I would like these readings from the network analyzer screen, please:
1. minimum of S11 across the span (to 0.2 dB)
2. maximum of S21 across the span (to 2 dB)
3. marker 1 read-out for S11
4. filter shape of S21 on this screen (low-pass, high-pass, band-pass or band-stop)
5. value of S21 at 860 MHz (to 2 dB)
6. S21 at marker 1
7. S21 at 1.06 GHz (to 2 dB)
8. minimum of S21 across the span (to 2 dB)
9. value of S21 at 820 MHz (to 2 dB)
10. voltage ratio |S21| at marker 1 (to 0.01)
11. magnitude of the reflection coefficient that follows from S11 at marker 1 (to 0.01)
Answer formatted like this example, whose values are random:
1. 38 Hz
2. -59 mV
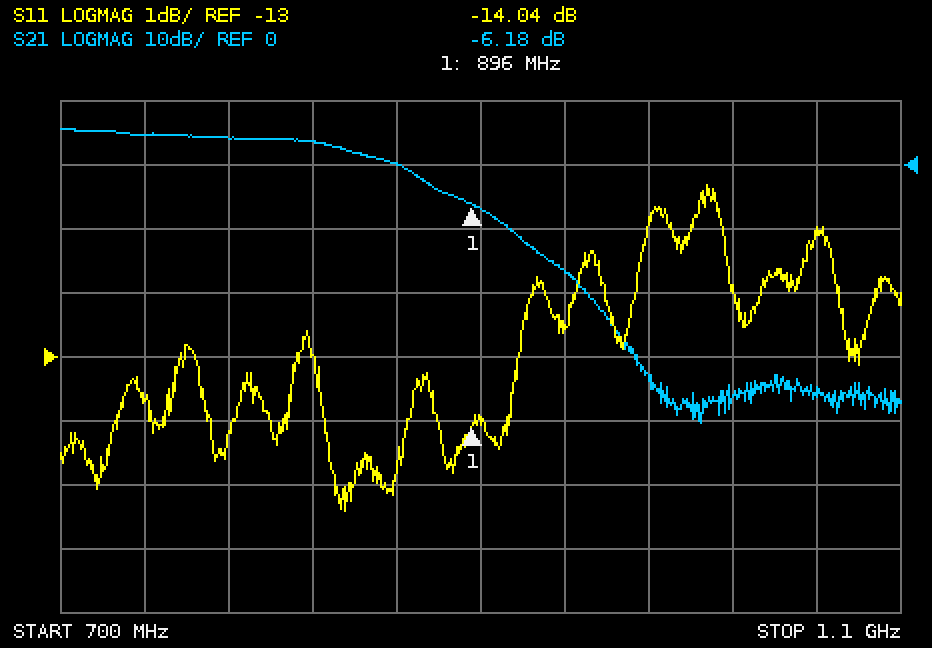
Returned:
1. -15.4 dB
2. 6 dB
3. -14.04 dB
4. low-pass
5. 0 dB
6. -6.18 dB
7. -36 dB
8. -40 dB
9. 4 dB
10. 0.49
11. 0.20
